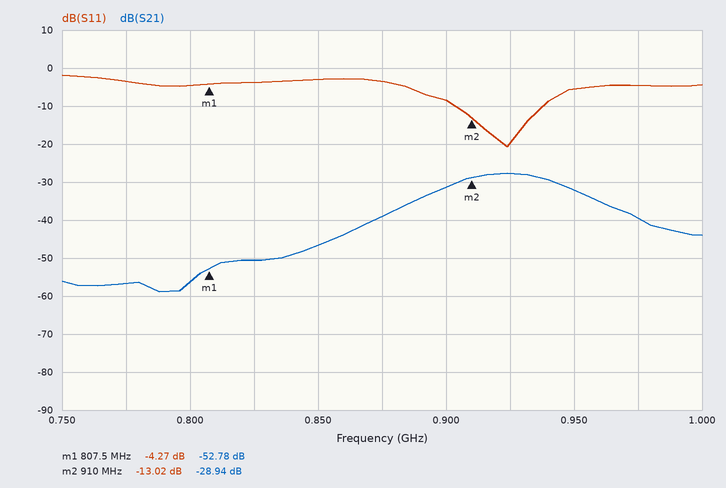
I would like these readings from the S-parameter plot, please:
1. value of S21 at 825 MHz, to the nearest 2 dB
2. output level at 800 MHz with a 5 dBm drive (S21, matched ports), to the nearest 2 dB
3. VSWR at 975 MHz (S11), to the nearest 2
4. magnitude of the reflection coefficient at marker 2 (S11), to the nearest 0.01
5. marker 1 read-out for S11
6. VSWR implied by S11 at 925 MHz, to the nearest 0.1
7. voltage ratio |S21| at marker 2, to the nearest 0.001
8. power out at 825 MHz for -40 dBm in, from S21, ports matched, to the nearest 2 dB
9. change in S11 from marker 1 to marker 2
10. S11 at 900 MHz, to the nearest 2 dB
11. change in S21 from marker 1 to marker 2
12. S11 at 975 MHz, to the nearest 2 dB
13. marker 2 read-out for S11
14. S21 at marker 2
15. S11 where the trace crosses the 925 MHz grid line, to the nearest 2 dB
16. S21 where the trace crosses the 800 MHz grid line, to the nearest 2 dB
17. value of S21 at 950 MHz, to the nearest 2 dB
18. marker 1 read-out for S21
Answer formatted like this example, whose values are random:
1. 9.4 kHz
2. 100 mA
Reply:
1. -50 dB
2. -52 dBm
3. 4
4. 0.22
5. -4.27 dB
6. 1.2
7. 0.036
8. -90 dBm
9. -8.75 dB
10. -8 dB
11. 23.84 dB
12. -4 dB
13. -13.02 dB
14. -28.94 dB
15. -20 dB
16. -56 dB
17. -32 dB
18. -52.78 dB
